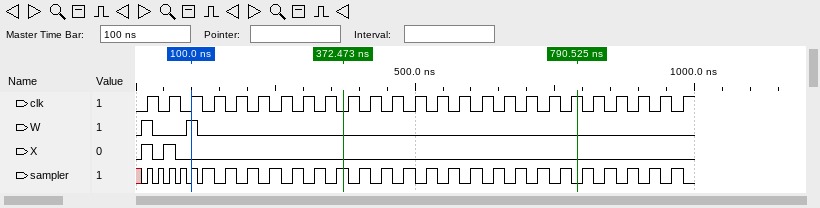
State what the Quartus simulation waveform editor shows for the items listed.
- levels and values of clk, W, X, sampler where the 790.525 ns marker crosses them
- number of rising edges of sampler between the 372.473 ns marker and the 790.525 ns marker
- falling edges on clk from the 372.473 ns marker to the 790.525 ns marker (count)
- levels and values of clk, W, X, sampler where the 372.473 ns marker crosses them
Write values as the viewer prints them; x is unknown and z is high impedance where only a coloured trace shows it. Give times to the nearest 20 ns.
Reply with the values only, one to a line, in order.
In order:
clk=1, W=0, X=0, sampler=0
10
10
clk=0, W=0, X=0, sampler=1
